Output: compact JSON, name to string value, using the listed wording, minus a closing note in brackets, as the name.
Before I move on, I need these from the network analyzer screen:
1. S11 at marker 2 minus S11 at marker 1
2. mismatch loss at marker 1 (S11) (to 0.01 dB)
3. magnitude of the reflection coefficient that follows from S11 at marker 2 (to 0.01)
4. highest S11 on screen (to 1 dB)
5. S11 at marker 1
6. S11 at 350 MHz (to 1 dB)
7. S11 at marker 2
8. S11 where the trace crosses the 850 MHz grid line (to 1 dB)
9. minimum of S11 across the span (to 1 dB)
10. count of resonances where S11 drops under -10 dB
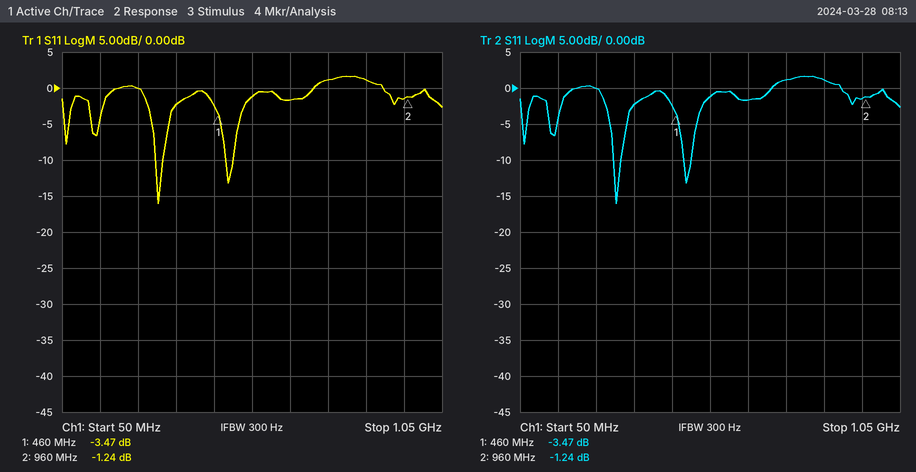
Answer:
{"S11 at marker 2 minus S11 at marker 1": "2.23 dB", "mismatch loss at marker 1 (S11)": "2.59 dB", "magnitude of the reflection coefficient that follows from S11 at marker 2": "0.87", "highest S11 on screen": "2 dB", "S11 at marker 1": "-3.47 dB", "S11 at 350 MHz": "-2 dB", "S11 at marker 2": "-1.24 dB", "S11 where the trace crosses the 850 MHz grid line": "1 dB", "minimum of S11 across the span": "-16 dB", "count of resonances where S11 drops under -10 dB": "2"}
